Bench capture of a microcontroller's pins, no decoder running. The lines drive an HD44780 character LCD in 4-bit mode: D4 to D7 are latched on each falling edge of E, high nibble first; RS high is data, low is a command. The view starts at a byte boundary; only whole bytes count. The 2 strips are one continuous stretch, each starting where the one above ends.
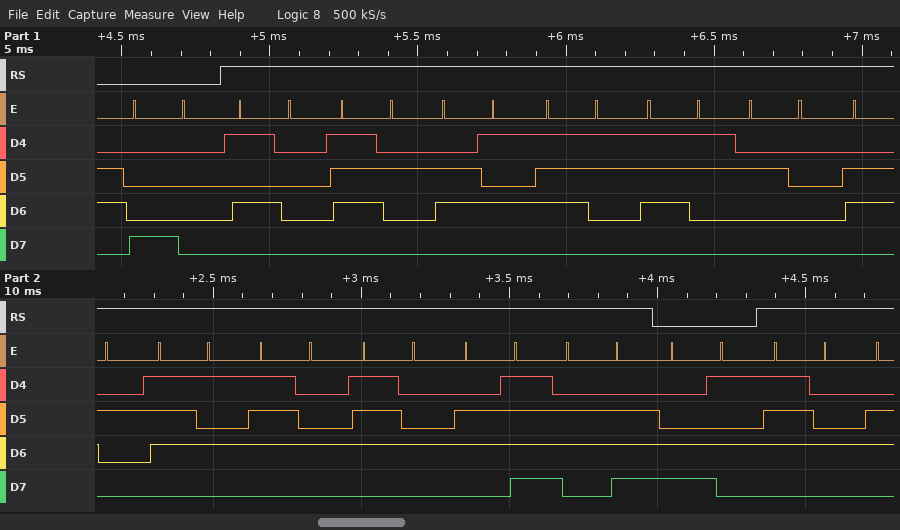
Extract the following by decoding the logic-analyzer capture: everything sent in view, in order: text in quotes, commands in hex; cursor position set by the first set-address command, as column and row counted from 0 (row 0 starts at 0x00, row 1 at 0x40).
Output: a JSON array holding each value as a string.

["0x80 \"Press button\" 0xC5 \"t\"", "column 0, row 0"]
